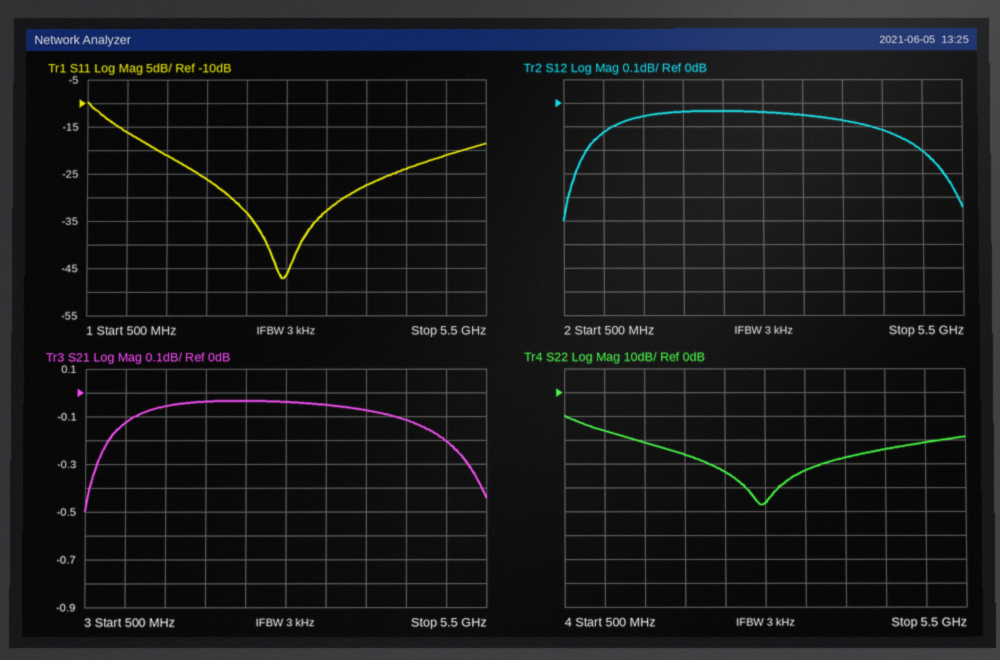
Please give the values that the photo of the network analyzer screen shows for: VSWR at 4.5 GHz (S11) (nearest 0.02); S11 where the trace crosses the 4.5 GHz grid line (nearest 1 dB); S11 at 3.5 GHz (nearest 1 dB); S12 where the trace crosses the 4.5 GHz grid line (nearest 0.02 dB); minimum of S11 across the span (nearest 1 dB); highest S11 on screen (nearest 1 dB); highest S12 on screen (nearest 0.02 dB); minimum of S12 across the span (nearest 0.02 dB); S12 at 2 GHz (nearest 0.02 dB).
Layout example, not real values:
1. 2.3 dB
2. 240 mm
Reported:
1. 1.14
2. -24 dB
3. -33 dB
4. -0.12 dB
5. -47 dB
6. -10 dB
7. -0.04 dB
8. -0.50 dB
9. -0.04 dB
